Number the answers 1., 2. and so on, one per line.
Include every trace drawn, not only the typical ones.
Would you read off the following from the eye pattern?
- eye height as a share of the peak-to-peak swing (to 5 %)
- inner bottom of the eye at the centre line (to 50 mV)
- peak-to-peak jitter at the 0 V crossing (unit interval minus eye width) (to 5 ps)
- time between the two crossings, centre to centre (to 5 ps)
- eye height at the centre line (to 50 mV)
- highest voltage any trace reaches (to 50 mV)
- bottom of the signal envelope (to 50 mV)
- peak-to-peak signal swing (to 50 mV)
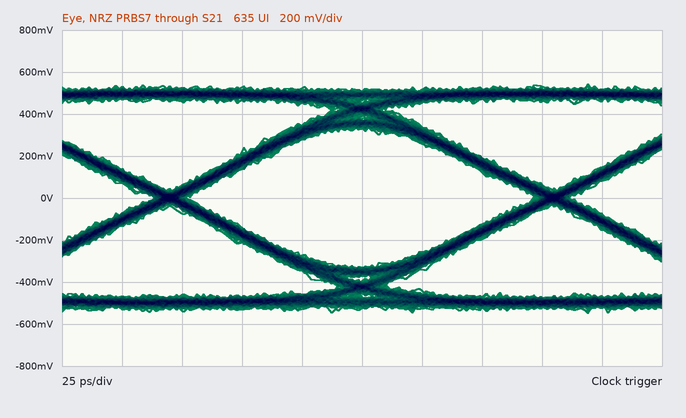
1. 60 %
2. -350 mV
3. 15 ps
4. 160 ps
5. 650 mV
6. 550 mV
7. -550 mV
8. 1.10 V
